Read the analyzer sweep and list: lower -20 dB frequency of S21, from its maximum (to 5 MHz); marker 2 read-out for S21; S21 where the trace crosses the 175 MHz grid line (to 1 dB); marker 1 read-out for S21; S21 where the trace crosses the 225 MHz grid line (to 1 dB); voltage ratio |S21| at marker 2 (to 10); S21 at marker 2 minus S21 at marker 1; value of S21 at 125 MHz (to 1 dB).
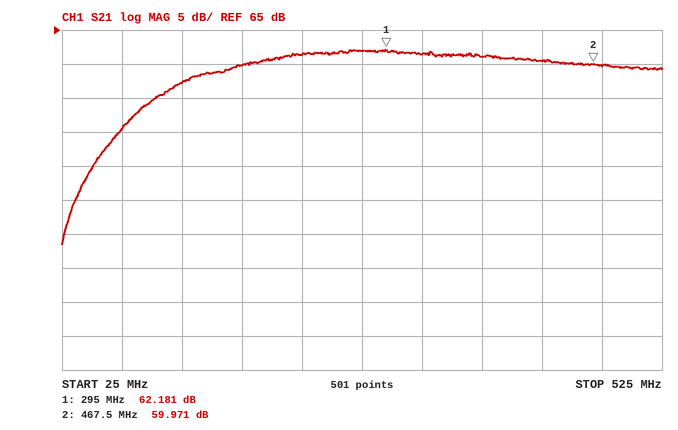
40 MHz
59.971 dB
60 dB
62.181 dB
61 dB
1000
-2.210 dB
57 dB
